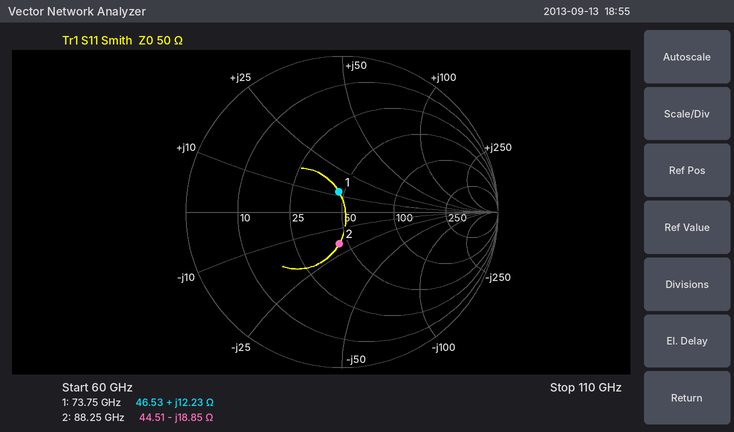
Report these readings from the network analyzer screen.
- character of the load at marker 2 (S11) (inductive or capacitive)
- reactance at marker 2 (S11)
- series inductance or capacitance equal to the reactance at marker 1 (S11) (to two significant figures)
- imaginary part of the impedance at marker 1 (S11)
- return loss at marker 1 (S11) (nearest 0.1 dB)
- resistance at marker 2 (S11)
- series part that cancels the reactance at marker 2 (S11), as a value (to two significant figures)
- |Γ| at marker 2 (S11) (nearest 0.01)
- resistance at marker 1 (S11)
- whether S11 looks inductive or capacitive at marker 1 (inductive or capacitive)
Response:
capacitive
-18.85 Ω
26 pH
+12.23 Ω
17.7 dB
44.51 Ω
34 pH
0.20
46.53 Ω
inductive
